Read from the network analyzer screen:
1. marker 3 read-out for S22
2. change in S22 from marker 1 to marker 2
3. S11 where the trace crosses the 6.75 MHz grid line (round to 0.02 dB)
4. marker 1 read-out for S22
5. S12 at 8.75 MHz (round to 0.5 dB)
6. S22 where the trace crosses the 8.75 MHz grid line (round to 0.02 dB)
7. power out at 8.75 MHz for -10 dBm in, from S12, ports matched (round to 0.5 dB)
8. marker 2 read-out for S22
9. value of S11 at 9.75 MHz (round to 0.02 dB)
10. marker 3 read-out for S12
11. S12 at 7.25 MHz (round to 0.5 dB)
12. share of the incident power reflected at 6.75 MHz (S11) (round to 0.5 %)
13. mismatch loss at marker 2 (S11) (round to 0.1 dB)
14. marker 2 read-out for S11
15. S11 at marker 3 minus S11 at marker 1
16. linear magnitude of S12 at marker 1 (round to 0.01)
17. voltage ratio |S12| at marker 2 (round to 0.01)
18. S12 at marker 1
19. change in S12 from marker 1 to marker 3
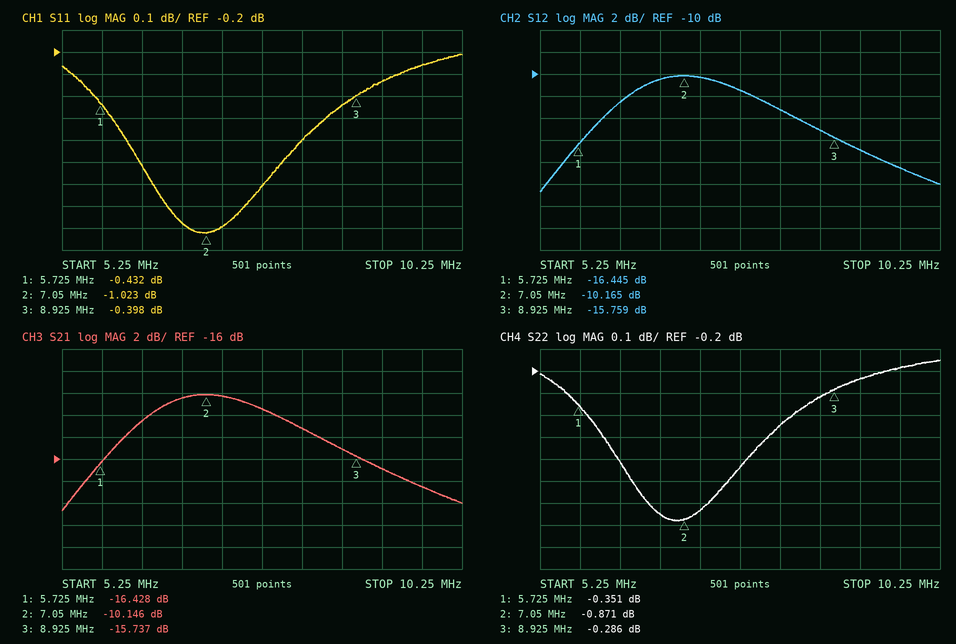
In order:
-0.286 dB
-0.520 dB
-0.98 dB
-0.351 dB
-15.0 dB
-0.32 dB
-25.0 dBm
-0.871 dB
-0.26 dB
-15.759 dB
-10.5 dB
80.0 %
6.8 dB
-1.023 dB
0.034 dB
0.15
0.31
-16.445 dB
0.686 dB
